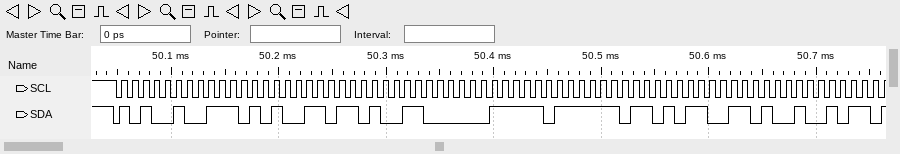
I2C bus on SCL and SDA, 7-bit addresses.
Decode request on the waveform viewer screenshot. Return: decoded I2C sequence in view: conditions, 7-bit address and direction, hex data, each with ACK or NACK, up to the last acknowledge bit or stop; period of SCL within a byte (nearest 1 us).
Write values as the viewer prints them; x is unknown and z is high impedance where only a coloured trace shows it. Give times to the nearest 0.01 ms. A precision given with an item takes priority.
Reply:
start, address 52 write NACK, D4 NACK, B4 NACK, 81 NACK, EF NACK, B5 NACK, 34 NACK
10 us
